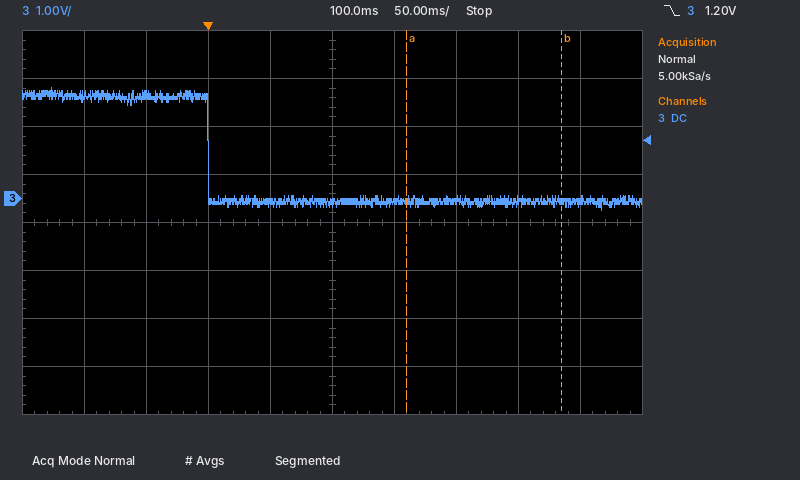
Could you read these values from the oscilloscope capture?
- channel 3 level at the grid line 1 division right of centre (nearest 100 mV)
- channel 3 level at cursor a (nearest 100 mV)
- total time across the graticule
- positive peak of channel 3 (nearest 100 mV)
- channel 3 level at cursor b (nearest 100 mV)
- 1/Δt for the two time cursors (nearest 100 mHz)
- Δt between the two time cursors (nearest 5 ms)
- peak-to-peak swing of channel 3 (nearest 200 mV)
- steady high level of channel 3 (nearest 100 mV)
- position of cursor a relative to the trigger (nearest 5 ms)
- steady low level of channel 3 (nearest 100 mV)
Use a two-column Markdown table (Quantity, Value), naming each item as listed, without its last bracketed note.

| Quantity | Value |
|---|---|
| channel 3 level at the grid line 1 division right of centre | -100 mV |
| channel 3 level at cursor a | 0.0 V |
| total time across the graticule | 500 ms |
| positive peak of channel 3 | 2.3 V |
| channel 3 level at cursor b | 0.0 V |
| 1/Δt for the two time cursors | 8.0 Hz |
| Δt between the two time cursors | 125 ms |
| peak-to-peak swing of channel 3 | 2.6 V |
| steady high level of channel 3 | 2.1 V |
| position of cursor a relative to the trigger | +160 ms |
| steady low level of channel 3 | -100 mV |
